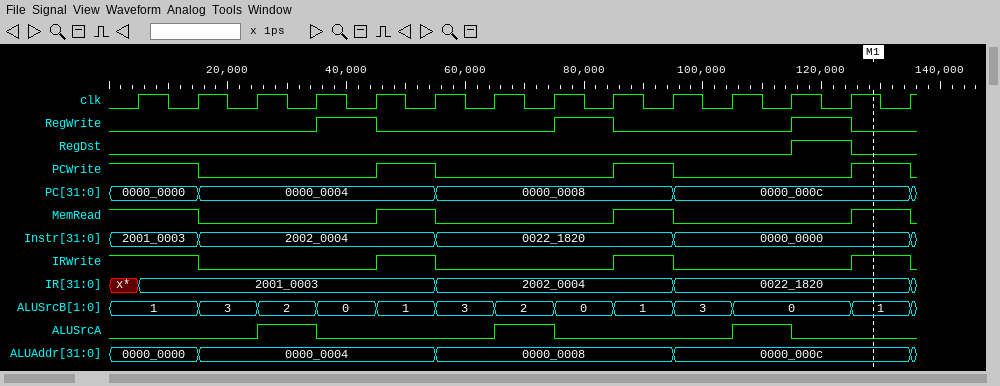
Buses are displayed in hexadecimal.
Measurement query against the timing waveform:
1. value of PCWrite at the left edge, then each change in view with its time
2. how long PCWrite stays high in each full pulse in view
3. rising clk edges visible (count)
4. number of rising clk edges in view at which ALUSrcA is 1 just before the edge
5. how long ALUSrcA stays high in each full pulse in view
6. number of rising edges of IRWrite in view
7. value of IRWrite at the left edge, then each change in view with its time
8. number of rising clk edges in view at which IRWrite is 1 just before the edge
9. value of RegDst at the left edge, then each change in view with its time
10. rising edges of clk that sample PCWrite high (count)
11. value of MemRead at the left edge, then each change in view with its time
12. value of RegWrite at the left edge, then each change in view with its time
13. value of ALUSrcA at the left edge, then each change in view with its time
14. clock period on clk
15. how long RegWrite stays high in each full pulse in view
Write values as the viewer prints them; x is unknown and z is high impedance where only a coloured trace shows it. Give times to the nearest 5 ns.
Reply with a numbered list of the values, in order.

1. 1, 0 at 15 ns, 1 at 45 ns, 0 at 55 ns, 1 at 85 ns, 0 at 95 ns, 1 at 125 ns, 0 at 135 ns
2. 10 ns, 10 ns, 10 ns
3. 14
4. 3
5. 10 ns, 10 ns, 10 ns
6. 3
7. 1, 0 at 15 ns, 1 at 45 ns, 0 at 55 ns, 1 at 85 ns, 0 at 95 ns, 1 at 125 ns, 0 at 135 ns
8. 5
9. 0, 1 at 115 ns, 0 at 125 ns
10. 5
11. 1, 0 at 15 ns, 1 at 45 ns, 0 at 55 ns, 1 at 85 ns, 0 at 95 ns, 1 at 125 ns, 0 at 135 ns
12. 0, 1 at 35 ns, 0 at 45 ns, 1 at 75 ns, 0 at 85 ns, 1 at 115 ns, 0 at 125 ns
13. 0, 1 at 25 ns, 0 at 35 ns, 1 at 65 ns, 0 at 75 ns, 1 at 105 ns, 0 at 115 ns
14. 10 ns
15. 10 ns, 10 ns, 10 ns
